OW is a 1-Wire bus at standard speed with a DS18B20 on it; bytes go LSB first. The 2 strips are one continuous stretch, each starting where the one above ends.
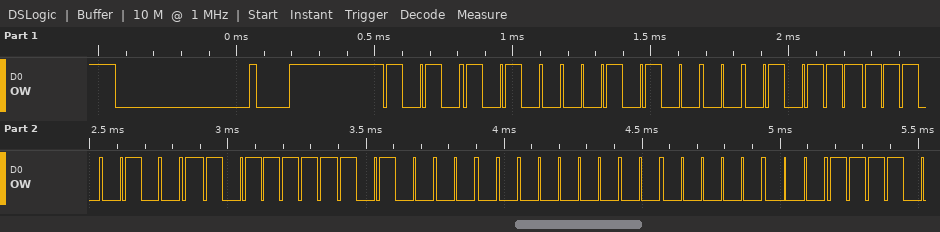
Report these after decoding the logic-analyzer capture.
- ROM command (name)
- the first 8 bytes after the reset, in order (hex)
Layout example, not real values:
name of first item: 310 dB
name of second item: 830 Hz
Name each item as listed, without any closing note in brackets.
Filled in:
ROM command: Match ROM
the first 8 bytes after the reset, in order: 55 28 E8 27 FB 05 00 00
